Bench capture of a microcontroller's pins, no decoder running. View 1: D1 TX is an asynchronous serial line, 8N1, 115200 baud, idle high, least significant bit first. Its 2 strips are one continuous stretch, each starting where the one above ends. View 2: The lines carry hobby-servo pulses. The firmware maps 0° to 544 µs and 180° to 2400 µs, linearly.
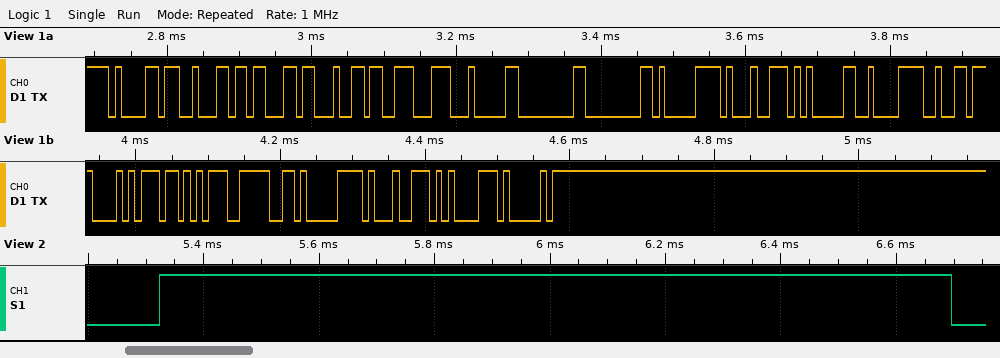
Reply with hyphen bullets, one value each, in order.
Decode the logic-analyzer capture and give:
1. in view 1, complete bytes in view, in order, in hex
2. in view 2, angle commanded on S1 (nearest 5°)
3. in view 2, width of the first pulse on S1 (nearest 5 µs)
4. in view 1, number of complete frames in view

- 0x61 0x62 0x63 0x64 0x8E 0x04 0x00 0x00 0xC1 0x91 0x05 0xC2 0xB2 0xA8 0xAB 0x3E 0xC1 0x91 0x85 0x41
- 80°
- 1370 µs
- 20
